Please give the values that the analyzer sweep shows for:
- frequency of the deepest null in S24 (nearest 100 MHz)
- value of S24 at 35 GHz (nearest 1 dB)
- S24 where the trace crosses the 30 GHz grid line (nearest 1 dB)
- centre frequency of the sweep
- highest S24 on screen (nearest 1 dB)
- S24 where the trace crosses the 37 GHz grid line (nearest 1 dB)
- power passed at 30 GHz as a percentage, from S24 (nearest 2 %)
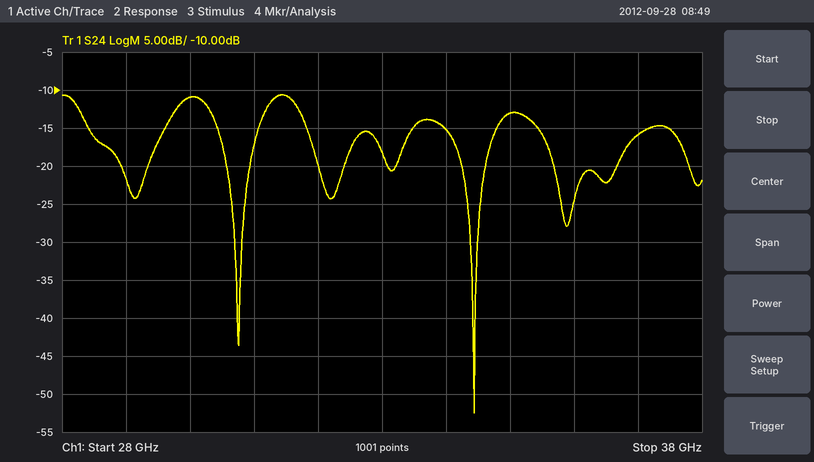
34.4 GHz
-13 dB
-11 dB
33 GHz
-11 dB
-16 dB
8 %
